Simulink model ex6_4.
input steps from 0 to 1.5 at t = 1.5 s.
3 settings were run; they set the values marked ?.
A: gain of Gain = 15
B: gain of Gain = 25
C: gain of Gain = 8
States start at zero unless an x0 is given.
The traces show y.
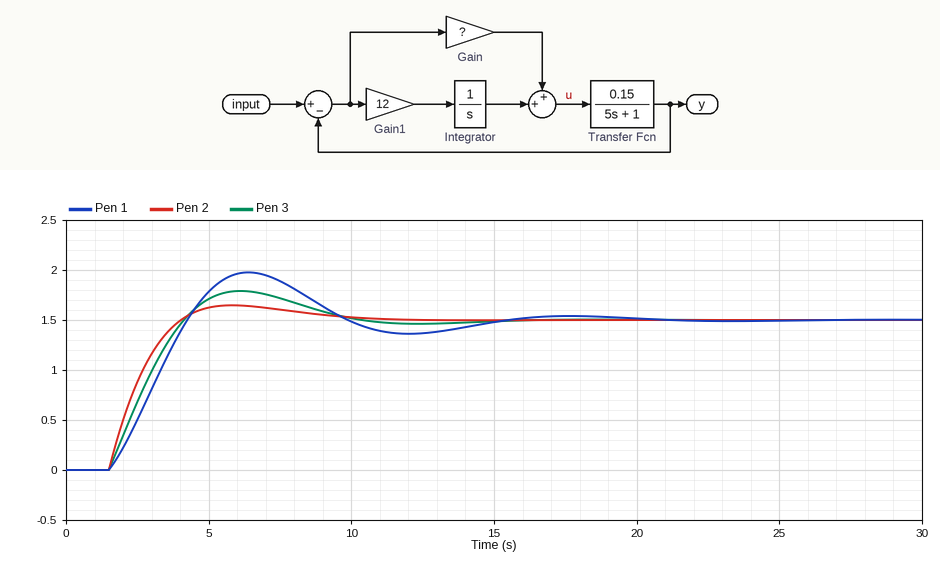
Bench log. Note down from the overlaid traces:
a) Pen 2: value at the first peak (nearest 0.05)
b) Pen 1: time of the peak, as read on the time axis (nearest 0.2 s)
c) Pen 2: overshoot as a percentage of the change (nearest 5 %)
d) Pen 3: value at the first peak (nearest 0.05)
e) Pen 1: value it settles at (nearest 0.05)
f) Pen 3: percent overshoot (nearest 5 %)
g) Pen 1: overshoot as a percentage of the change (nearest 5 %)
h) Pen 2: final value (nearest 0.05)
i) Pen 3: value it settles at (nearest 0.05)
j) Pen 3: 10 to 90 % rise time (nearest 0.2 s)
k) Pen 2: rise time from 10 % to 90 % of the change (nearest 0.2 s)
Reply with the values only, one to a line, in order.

1.65
6.4 s
10 %
1.80
1.50
20 %
30 %
1.50
1.50
2.0 s
1.8 s
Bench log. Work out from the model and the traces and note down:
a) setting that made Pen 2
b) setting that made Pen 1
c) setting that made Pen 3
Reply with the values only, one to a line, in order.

B
C
A
